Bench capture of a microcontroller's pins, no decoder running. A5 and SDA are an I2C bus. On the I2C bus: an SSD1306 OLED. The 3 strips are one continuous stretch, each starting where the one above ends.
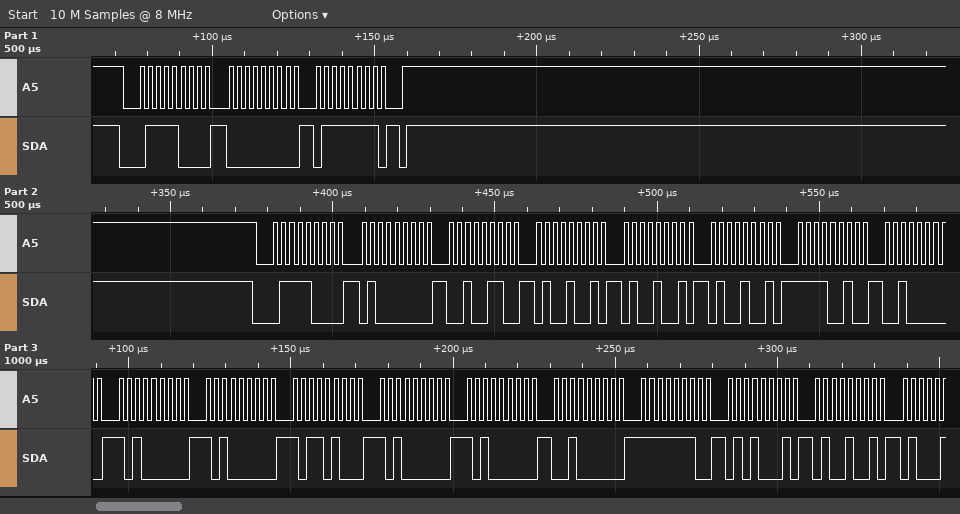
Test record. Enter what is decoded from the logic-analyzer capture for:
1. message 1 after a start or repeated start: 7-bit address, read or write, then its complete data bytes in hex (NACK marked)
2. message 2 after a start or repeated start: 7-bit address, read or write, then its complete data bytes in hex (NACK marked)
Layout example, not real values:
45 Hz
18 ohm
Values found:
0x3C write: 00 7F
0x3C write: 40 26 49 49 49 F2 20 A0 A0 B4 A0 A0 20 FE 51 49
